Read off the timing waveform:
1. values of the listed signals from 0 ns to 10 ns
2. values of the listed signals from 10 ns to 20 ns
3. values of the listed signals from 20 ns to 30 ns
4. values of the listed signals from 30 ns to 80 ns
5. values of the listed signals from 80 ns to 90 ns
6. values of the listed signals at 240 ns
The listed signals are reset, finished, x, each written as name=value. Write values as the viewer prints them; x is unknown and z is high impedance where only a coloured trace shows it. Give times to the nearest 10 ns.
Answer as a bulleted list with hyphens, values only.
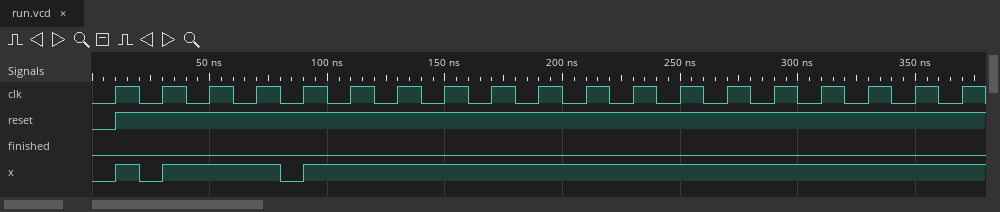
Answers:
- reset=0, finished=0, x=0
- reset=1, finished=0, x=1
- reset=1, finished=0, x=0
- reset=1, finished=0, x=1
- reset=1, finished=0, x=0
- reset=1, finished=0, x=1
